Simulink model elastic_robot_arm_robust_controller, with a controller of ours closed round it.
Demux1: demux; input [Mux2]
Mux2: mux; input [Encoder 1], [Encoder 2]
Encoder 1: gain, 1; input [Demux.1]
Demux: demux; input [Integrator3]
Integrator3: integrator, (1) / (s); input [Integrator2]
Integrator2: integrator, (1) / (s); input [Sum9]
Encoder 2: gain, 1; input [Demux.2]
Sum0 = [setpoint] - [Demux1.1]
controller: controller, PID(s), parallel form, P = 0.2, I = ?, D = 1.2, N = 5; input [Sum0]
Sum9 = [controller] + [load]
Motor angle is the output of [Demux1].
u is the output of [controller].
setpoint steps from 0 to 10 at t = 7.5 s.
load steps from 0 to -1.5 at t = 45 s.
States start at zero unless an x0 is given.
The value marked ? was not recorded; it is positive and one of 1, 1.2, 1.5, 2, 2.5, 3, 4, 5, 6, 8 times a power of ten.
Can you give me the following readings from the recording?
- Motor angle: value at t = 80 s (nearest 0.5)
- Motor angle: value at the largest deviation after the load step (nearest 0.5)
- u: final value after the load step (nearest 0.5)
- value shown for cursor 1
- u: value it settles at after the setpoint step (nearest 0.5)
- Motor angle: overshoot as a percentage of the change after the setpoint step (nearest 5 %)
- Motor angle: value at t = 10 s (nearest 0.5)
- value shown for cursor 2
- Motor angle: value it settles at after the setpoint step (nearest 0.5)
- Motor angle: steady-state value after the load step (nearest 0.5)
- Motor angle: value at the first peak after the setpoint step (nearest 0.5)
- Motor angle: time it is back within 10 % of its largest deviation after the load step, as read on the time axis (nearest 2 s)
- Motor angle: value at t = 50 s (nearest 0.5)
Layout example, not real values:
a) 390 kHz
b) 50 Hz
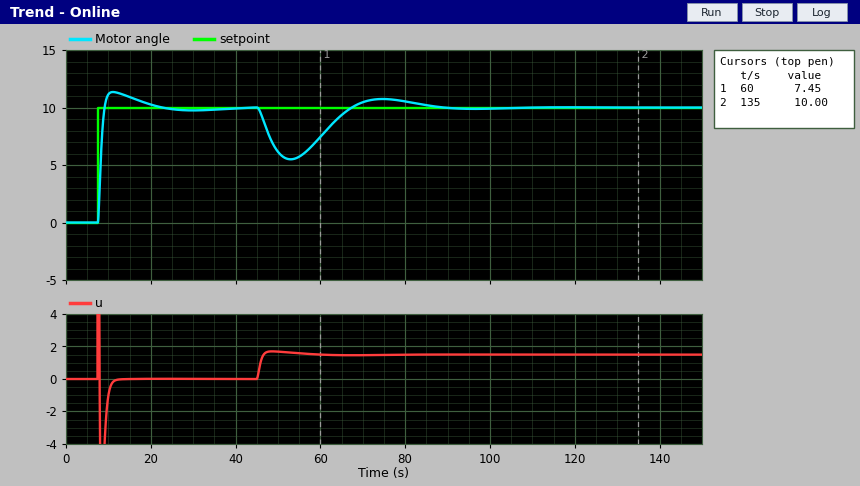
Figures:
a) 10.5
b) 5.5
c) 1.5
d) 7.45
e) 0.0
f) 15 %
g) 11.0
h) 10.00
i) 10.0
j) 10.0
k) 11.5
l) 82 s
m) 6.0
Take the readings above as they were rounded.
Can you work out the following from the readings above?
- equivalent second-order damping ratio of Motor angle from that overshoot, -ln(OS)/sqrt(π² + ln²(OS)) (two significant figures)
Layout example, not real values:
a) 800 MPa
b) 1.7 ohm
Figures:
a) 0.52
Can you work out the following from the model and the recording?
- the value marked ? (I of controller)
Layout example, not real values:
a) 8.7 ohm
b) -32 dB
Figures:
a) 0.03
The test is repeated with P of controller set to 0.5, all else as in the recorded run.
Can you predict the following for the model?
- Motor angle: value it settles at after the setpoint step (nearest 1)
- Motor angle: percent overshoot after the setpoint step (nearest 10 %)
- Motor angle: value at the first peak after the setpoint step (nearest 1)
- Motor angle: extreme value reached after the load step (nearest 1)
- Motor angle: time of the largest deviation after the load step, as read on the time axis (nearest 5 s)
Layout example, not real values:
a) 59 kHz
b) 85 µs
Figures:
a) 10
b) 20 %
c) 12
d) 7
e) 50 s
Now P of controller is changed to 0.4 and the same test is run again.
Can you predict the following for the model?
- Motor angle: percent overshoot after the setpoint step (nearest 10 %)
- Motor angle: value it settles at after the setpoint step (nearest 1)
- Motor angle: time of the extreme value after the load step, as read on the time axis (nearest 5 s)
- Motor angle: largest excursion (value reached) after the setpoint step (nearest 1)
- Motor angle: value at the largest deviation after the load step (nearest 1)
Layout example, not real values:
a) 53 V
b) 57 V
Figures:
a) 20 %
b) 10
c) 50 s
d) 12
e) 7
